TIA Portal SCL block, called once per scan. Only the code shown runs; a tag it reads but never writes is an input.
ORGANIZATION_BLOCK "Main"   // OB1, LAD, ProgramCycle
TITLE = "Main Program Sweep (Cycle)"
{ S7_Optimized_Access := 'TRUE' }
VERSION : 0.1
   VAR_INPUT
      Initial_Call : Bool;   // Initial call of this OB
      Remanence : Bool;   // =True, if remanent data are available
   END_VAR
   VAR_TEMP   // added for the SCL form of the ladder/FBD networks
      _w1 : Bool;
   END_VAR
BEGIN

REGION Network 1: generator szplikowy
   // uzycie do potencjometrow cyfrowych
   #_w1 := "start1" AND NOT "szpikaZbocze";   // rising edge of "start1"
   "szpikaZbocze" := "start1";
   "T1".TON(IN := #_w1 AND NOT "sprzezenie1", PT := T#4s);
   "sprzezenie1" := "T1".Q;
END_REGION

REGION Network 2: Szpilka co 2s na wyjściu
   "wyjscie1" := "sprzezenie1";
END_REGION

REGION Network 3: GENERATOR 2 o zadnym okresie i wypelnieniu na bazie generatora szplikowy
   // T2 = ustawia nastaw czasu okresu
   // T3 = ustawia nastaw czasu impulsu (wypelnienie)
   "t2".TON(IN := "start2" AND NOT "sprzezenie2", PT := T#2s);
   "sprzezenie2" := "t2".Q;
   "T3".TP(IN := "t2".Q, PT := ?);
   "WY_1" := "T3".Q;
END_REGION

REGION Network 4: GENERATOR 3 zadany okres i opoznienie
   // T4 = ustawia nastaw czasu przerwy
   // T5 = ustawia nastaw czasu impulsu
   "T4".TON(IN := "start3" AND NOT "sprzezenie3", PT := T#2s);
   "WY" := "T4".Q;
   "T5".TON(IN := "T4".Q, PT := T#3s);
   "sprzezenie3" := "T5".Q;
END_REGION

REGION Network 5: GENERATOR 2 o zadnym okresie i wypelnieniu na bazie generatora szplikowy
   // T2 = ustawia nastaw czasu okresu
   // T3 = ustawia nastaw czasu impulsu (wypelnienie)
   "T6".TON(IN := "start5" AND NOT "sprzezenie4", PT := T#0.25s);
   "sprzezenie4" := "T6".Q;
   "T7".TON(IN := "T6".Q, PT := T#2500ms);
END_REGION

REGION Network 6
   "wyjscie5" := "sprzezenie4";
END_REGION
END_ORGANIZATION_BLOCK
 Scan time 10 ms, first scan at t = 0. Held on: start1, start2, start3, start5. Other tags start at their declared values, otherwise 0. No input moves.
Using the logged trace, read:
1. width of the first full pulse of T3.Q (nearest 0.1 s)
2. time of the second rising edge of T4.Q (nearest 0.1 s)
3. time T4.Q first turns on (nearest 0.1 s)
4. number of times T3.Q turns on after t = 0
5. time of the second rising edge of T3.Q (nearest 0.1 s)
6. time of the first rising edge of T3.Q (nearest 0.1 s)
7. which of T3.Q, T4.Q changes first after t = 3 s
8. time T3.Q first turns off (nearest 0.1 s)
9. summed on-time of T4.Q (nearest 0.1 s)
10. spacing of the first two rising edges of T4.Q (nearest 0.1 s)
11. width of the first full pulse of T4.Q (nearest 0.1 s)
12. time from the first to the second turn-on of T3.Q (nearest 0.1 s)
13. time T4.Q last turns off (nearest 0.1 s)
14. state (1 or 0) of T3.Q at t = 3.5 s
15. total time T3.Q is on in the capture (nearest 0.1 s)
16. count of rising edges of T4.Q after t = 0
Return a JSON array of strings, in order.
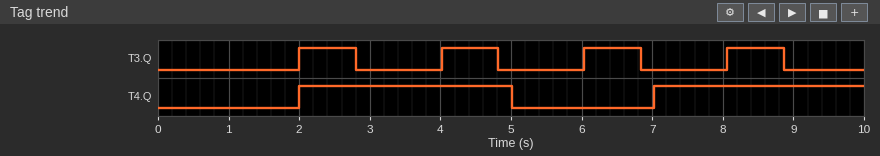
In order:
["0.8 s", "7.0 s", "2.0 s", "4", "4.0 s", "2.0 s", "T3.Q", "2.8 s", "6.0 s", "5.0 s", "3.0 s", "2.0 s", "5.0 s", "0", "3.2 s", "2"]
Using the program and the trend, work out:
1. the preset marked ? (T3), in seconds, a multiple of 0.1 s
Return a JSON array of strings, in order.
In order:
["0.8 s"]
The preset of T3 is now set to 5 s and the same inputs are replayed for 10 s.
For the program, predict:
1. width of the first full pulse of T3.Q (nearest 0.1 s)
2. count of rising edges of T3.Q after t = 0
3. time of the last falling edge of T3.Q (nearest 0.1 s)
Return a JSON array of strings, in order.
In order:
["5.0 s", "2", "7.0 s"]
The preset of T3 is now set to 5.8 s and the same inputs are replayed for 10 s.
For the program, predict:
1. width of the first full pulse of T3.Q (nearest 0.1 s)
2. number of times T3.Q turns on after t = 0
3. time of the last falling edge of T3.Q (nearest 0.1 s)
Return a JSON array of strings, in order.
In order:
["5.8 s", "2", "7.8 s"]
